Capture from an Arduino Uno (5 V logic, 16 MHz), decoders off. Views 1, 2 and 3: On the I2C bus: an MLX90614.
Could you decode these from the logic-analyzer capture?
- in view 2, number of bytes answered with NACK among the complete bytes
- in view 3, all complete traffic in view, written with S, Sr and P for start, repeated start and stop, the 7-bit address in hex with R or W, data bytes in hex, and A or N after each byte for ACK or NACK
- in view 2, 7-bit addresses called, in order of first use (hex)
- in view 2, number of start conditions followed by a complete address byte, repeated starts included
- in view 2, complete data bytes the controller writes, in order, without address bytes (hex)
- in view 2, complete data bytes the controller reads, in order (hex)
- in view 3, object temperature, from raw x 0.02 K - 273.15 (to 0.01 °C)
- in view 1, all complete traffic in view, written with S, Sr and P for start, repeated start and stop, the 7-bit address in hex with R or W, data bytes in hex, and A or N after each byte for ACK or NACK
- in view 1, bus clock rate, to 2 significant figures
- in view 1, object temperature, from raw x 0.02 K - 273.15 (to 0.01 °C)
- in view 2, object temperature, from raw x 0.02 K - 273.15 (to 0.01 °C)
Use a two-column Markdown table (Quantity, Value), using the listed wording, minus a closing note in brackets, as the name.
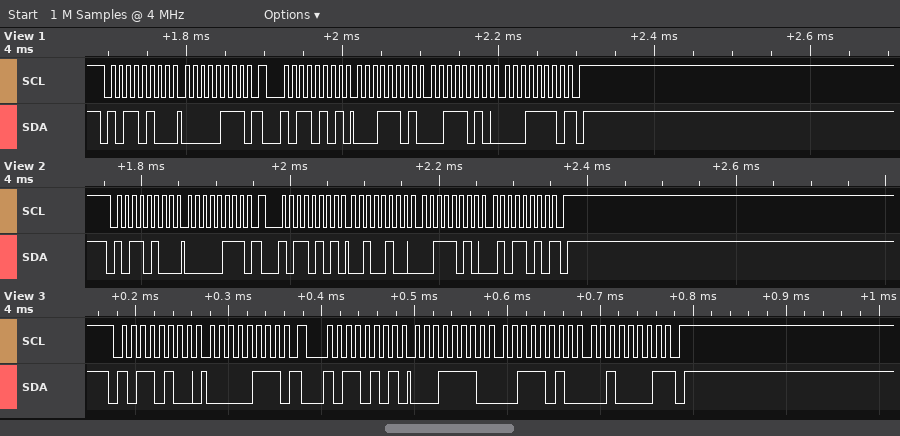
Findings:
| Quantity | Value |
|---|---|
| in view 2, number of bytes answered with NACK among the complete bytes | 1 |
| in view 3, all complete traffic in view, written with S, Sr and P for start, repeated start and stop, the 7-bit address in hex with R or W, data bytes in hex, and A or N after each byte for ACK or NACK | S 5AW A 07 A Sr 5AR A 1E A 3A A 21 N P |
| in view 2, 7-bit addresses called, in order of first use | 0x5A |
| in view 2, number of start conditions followed by a complete address byte, repeated starts included | 2 |
| in view 2, complete data bytes the controller writes, in order, without address bytes | 07 |
| in view 2, complete data bytes the controller reads, in order | 24 3A 5A |
| in view 3, object temperature, from raw x 0.02 K - 273.15 | 24.41 °C |
| in view 1, all complete traffic in view, written with S, Sr and P for start, repeated start and stop, the 7-bit address in hex with R or W, data bytes in hex, and A or N after each byte for ACK or NACK | S 5AW A 07 A Sr 5AR A 1D A 3A A 1E N P |
| in view 1, bus clock rate, to 2 significant figures | 100 kHz |
| in view 1, object temperature, from raw x 0.02 K - 273.15 | 24.39 °C |
| in view 2, object temperature, from raw x 0.02 K - 273.15 | 24.53 °C |
